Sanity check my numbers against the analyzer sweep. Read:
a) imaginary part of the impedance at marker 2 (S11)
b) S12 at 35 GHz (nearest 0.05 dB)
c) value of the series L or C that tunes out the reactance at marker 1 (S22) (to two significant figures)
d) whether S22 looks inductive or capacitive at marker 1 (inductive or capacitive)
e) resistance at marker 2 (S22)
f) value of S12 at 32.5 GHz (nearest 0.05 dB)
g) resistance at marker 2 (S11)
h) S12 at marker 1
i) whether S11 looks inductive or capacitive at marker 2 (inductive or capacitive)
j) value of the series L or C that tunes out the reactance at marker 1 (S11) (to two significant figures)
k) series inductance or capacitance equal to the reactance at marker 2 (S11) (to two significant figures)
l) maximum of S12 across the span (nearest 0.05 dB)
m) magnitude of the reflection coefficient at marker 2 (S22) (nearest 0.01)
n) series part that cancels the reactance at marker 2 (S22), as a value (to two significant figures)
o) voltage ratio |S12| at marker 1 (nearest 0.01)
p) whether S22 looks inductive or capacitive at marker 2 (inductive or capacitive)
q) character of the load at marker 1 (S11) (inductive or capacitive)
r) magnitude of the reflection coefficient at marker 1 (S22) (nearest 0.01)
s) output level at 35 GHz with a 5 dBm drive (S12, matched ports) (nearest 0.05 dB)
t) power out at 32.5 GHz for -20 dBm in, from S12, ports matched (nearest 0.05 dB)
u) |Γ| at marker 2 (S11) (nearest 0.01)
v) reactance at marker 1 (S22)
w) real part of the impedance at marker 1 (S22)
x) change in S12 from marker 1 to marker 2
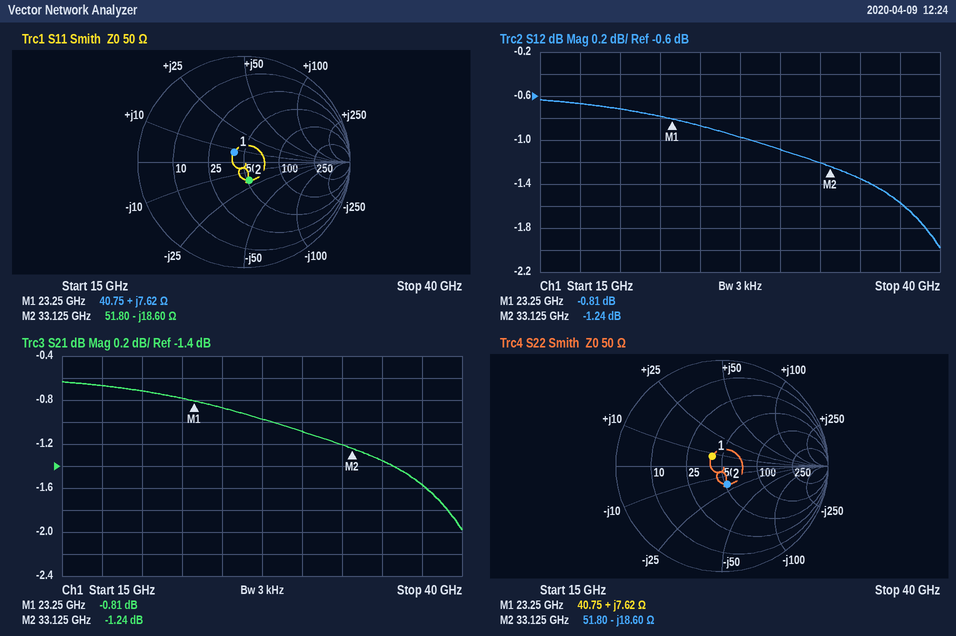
-18.60 Ω
-1.35 dB
900 fF
inductive
51.80 Ω
-1.20 dB
51.80 Ω
-0.81 dB
capacitive
900 fF
260 fF
-0.65 dB
0.18
89 pH
0.91
capacitive
inductive
0.13
3.65 dBm
-21.20 dBm
0.18
+7.62 Ω
40.75 Ω
-0.43 dB
